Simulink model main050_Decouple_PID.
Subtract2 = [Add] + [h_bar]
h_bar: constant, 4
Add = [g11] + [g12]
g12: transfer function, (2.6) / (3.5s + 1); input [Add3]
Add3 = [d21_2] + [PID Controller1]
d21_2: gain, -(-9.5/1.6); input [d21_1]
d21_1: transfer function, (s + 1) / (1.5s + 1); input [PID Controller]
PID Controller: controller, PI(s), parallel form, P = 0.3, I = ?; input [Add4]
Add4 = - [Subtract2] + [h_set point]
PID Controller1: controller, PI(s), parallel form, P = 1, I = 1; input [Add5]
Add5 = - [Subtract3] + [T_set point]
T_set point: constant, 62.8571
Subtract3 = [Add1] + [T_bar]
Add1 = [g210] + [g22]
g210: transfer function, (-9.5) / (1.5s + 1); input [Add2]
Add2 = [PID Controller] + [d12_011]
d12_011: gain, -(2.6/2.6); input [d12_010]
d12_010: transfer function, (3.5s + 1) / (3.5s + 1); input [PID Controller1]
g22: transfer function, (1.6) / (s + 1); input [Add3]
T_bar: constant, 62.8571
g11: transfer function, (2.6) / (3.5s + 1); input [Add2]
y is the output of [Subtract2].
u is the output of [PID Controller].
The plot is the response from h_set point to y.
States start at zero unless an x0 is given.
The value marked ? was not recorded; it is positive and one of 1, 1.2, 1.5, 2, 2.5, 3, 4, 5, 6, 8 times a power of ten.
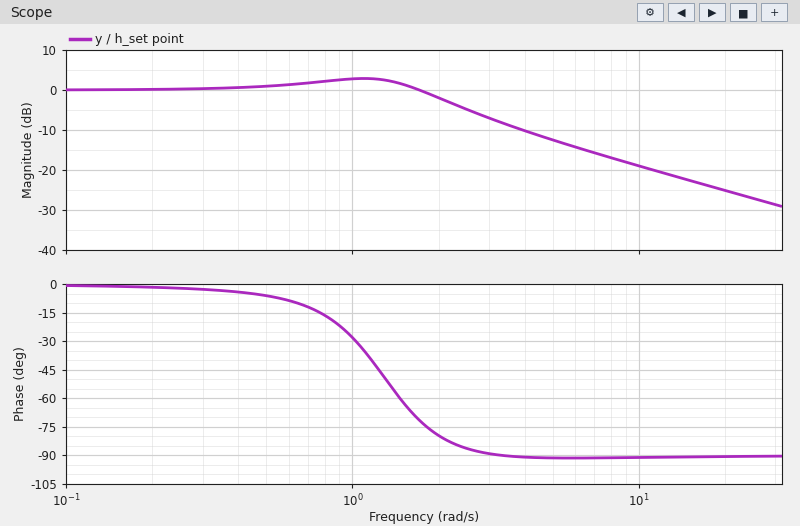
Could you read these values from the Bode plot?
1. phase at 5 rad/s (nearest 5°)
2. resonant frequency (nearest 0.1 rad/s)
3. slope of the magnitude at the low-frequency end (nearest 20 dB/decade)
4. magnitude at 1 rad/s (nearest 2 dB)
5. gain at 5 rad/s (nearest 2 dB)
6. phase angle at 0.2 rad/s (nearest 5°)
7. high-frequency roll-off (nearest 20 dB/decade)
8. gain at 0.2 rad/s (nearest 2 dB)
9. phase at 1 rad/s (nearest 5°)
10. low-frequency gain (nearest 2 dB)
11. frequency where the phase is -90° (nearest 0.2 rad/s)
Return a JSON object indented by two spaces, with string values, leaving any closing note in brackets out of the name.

{
  "phase at 5 rad/s": "-90°",
  "resonant frequency": "1.1 rad/s",
  "slope of the magnitude at the low-frequency end": "0 dB/decade",
  "magnitude at 1 rad/s": "2 dB",
  "gain at 5 rad/s": "-12 dB",
  "phase angle at 0.2 rad/s": "0°",
  "high-frequency roll-off": "-20 dB/decade",
  "gain at 0.2 rad/s": "0 dB",
  "phase at 1 rad/s": "-30°",
  "low-frequency gain": "0 dB",
  "frequency where the phase is -90°": "3.4 rad/s"
}
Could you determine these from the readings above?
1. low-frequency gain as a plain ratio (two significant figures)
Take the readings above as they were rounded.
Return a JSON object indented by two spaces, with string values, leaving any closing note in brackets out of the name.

{
  "low-frequency gain as a plain ratio": "1.0"
}
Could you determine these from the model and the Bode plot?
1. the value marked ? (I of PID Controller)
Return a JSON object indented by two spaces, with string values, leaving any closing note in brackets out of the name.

{
  "the value marked ?": "0.4"
}
